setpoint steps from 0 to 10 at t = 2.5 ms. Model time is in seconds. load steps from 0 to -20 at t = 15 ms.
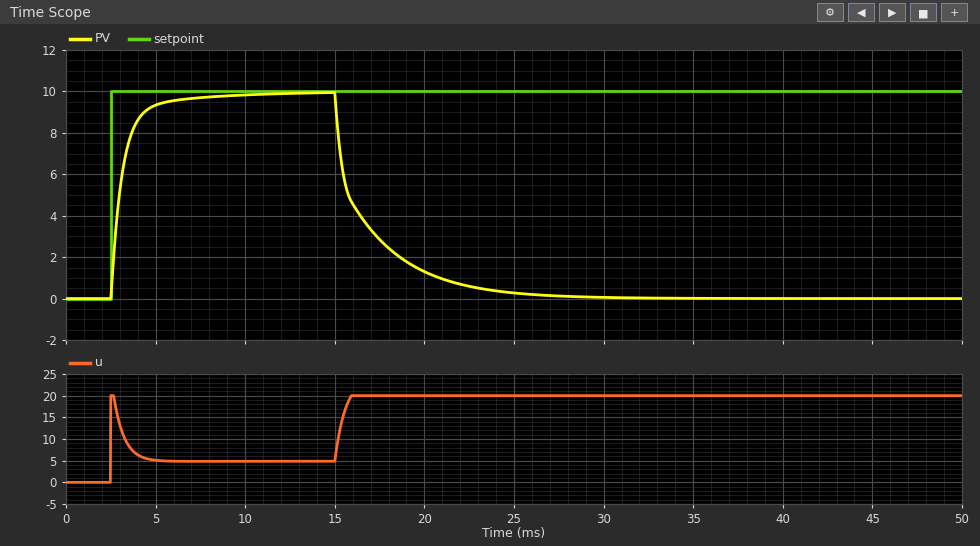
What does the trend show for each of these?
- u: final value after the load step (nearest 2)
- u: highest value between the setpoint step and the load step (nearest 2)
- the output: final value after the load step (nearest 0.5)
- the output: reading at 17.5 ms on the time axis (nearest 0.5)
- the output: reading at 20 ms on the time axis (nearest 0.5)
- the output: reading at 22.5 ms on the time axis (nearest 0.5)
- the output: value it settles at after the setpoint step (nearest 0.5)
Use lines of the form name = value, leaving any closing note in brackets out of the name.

u: final value after the load step = 20
u: highest value between the setpoint step and the load step = 20
the output: final value after the load step = 0.0
the output: reading at 17.5 ms on the time axis = 3.0
the output: reading at 20 ms on the time axis = 1.5
the output: reading at 22.5 ms on the time axis = 0.5
the output: value it settles at after the setpoint step = 10.0
